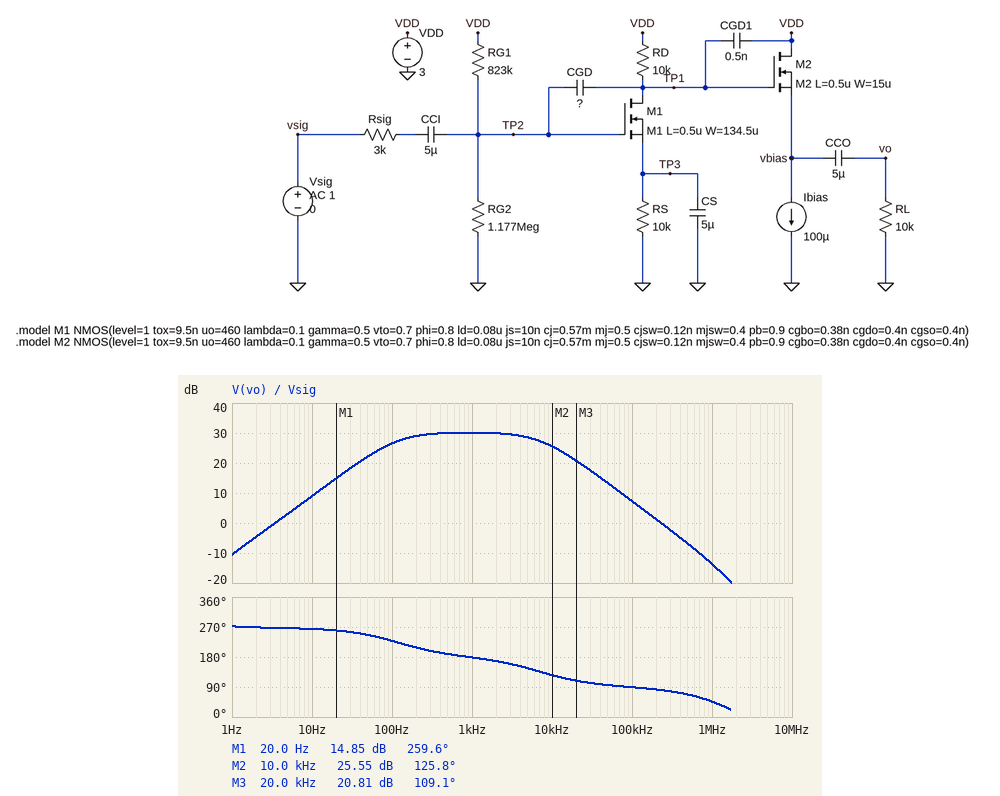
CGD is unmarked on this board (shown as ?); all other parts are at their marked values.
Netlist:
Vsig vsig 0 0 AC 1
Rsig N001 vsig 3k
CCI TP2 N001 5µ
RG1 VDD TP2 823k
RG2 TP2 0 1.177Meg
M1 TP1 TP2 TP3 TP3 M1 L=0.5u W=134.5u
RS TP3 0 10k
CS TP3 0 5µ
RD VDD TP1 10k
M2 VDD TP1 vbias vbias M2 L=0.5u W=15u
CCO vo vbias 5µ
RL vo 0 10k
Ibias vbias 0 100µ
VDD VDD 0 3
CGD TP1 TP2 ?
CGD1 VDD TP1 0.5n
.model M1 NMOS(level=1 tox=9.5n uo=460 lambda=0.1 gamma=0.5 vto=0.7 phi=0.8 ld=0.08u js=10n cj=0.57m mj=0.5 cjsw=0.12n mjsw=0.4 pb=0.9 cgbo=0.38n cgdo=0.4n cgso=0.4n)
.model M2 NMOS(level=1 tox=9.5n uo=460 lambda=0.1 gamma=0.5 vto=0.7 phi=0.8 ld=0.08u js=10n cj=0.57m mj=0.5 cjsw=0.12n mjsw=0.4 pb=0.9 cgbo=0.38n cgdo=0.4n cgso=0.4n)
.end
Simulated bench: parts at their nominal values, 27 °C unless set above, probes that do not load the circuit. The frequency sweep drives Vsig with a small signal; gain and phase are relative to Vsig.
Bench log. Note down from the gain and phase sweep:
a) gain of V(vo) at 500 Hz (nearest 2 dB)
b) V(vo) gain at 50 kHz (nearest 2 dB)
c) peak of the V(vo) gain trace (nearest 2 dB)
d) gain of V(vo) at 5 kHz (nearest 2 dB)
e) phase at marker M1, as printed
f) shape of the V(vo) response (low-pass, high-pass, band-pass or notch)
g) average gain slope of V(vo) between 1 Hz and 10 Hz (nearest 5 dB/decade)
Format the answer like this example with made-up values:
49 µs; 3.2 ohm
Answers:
30 dB; 14 dB; 30 dB; 28 dB; 259.6 deg; band-pass; 20 dB/decade
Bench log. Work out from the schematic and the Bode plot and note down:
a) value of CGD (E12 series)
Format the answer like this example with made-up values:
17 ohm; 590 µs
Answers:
150 pF
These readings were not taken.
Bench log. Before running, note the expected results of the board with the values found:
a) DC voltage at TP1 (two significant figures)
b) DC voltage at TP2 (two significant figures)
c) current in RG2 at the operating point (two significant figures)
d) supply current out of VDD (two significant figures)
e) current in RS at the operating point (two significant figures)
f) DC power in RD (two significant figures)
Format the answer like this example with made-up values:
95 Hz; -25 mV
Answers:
2.0 V; 1.8 V; 1.5 µA; 200 µA; 100 µA; 100 µW
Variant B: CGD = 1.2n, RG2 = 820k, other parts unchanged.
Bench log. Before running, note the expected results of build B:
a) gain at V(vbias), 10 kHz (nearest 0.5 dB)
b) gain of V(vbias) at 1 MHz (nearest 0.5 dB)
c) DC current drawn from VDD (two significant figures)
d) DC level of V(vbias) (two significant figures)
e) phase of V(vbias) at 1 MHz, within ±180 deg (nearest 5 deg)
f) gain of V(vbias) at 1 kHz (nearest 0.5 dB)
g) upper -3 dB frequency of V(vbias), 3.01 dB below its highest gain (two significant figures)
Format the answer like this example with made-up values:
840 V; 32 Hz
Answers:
11.0 dB; -23.5 dB; 180 µA; 1.4 V; -15 deg; 27.5 dB; 1.3 kHz
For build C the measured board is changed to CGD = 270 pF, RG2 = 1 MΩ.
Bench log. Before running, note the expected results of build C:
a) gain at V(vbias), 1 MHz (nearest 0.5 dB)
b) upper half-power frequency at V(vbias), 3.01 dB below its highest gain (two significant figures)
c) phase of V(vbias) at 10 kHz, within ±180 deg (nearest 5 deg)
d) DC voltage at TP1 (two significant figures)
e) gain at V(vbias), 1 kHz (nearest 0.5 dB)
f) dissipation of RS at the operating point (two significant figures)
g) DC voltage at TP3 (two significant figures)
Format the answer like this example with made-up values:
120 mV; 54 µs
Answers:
-18.0 dB; 4.7 kHz; 115 deg; 2.1 V; 29.5 dB; 80 µW; 900 mV
